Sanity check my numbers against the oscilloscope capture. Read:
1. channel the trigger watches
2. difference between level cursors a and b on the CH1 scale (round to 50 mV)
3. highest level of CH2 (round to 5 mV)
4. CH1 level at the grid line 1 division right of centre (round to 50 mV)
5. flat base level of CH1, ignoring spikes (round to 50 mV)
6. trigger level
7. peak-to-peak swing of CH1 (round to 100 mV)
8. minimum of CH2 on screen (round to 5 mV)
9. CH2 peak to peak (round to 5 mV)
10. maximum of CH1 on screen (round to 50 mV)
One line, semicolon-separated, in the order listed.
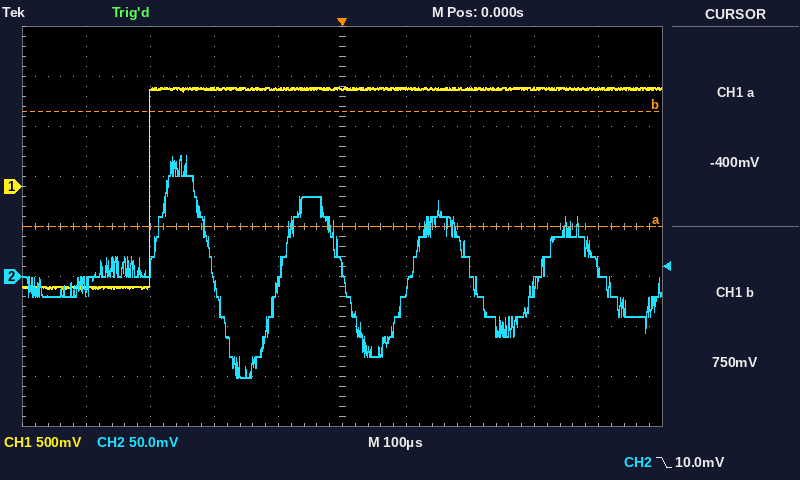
CH2; 1.15 V; 120 mV; 1.00 V; -1.00 V; 10.0 mV; 2.00 V; -100 mV; 220 mV; 1.00 V
